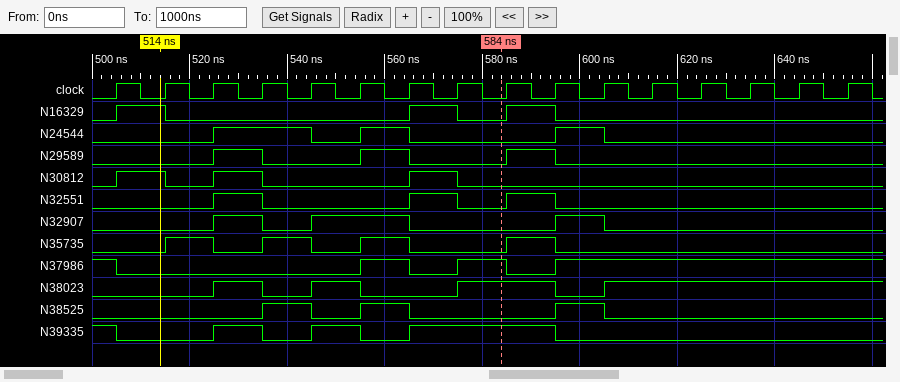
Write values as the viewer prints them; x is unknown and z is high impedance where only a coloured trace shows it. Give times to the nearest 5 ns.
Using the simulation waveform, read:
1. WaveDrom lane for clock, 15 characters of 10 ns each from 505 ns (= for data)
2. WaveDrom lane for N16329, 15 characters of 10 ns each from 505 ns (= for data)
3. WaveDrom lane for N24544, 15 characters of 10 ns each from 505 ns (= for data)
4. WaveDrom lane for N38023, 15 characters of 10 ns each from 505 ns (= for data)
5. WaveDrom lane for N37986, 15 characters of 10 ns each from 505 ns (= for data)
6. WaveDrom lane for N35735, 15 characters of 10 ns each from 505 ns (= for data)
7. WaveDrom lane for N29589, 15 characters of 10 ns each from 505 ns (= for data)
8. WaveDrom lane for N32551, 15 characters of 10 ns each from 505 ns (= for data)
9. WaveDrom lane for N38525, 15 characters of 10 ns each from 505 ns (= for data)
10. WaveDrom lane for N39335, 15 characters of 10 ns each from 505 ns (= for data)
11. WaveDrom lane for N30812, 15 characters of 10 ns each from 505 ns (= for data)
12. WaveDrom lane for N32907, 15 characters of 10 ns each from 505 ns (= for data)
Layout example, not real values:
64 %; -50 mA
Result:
{name: 'clock', wave: 'p..............'}; {name: 'N16329', wave: '10....1010.....'}; {name: 'N24544', wave: '0.1.010..10....'}; {name: 'N38023', wave: '0.1010.1.01....'}; {name: 'N37986', wave: '0....10101.....'}; {name: 'N35735', wave: '0101010.10.....'}; {name: 'N29589', wave: '0.10.10.10.....'}; {name: 'N32551', wave: '0.10..1010.....'}; {name: 'N38525', wave: '0..1010..10....'}; {name: 'N39335', wave: '0.10101..0.....'}; {name: 'N30812', wave: '1010..10.......'}; {name: 'N32907', wave: '0.101.0..10....'}
